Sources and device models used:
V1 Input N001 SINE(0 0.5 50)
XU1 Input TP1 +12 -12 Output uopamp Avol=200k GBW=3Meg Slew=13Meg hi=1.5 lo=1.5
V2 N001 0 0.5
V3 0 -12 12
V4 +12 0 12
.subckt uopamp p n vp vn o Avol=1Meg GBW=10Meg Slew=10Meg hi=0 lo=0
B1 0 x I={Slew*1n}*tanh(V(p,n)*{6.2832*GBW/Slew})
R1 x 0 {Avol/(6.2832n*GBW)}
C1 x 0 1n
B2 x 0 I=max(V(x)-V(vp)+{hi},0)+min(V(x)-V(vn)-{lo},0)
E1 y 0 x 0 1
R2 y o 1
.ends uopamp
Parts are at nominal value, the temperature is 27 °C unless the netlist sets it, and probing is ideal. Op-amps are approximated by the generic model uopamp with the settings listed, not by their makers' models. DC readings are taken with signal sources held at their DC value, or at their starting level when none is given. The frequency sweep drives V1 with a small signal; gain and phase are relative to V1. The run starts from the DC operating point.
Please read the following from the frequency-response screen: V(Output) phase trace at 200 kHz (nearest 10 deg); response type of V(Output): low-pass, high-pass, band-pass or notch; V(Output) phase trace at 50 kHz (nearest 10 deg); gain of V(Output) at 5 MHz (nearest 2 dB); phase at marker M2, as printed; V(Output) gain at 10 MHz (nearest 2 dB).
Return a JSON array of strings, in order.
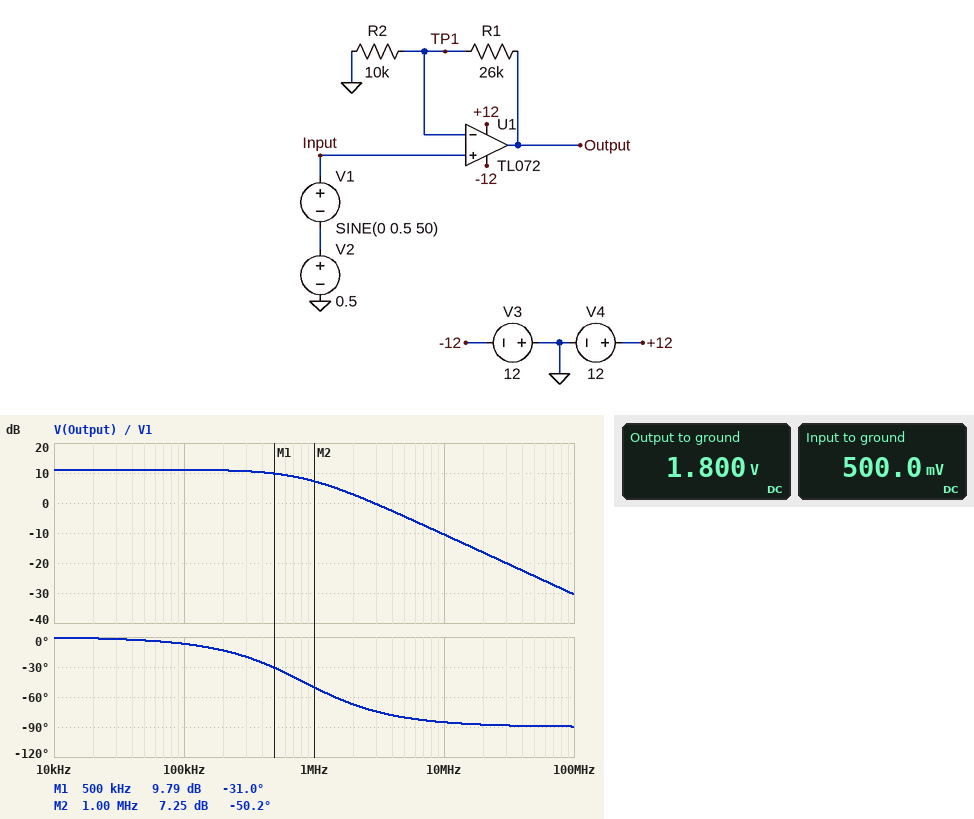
["-10 deg", "low-pass", "0 deg", "-4 dB", "-50.2 deg", "-10 dB"]
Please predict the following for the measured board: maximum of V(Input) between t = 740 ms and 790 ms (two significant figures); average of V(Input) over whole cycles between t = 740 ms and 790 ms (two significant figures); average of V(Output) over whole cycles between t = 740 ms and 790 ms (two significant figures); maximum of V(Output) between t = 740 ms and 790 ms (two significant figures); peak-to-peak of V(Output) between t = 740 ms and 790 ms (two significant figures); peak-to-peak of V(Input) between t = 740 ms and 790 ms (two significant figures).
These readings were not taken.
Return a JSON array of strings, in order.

["1.0 V", "500 mV", "1.8 V", "3.6 V", "3.6 V", "1.0 V"]
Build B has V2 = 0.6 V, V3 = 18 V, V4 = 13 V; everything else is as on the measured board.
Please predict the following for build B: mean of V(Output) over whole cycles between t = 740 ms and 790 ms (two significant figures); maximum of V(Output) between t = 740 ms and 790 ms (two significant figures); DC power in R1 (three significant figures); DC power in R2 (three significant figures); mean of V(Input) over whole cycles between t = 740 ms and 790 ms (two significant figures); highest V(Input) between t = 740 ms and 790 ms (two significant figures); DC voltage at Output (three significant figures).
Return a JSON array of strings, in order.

["2.2 V", "4.0 V", "93.6 µW", "36.0 µW", "600 mV", "1.1 V", "2.16 V"]
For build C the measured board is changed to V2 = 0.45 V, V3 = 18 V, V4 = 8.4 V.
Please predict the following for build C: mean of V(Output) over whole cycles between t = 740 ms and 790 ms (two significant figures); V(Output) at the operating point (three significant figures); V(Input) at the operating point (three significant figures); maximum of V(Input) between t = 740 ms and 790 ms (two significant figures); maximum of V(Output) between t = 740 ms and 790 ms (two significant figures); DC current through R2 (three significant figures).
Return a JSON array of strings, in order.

["1.6 V", "1.62 V", "450 mV", "950 mV", "3.4 V", "45.0 µA"]
